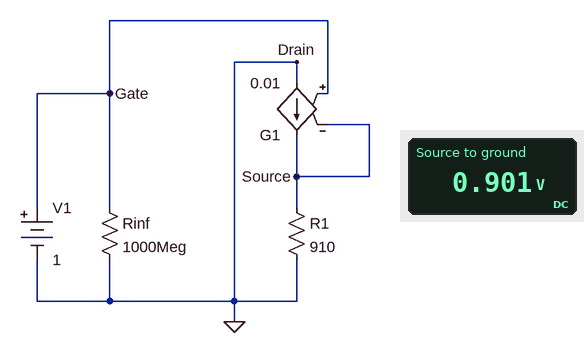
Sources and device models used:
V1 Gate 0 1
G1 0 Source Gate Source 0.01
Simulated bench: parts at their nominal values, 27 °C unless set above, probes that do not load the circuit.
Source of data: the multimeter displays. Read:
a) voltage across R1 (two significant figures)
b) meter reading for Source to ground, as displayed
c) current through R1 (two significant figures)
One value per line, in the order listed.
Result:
900 mV
0.901 V
990 µA
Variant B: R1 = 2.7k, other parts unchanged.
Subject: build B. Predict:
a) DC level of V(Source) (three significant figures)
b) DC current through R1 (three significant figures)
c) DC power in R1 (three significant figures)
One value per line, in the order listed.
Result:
964 mV
357 µA
344 µW
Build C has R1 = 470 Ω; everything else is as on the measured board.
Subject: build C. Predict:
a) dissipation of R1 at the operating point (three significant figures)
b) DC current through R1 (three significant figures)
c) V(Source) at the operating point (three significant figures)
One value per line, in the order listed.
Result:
1.45 mW
1.75 mA
825 mV
